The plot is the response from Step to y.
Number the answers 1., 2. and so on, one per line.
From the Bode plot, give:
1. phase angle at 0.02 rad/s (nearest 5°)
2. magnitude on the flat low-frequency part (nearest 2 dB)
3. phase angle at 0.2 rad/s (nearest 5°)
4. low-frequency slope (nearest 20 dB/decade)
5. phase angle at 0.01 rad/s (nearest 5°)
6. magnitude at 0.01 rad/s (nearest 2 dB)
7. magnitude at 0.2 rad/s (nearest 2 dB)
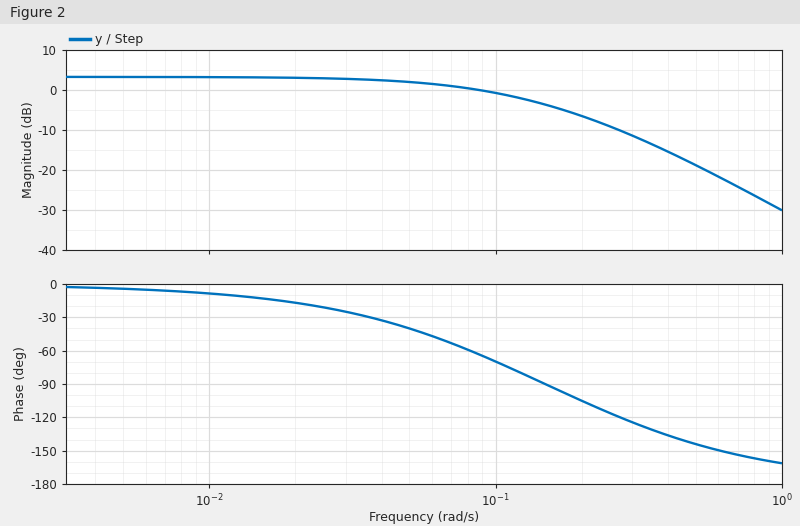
1. -15°
2. 4 dB
3. -105°
4. 0 dB/decade
5. -10°
6. 4 dB
7. -6 dB
